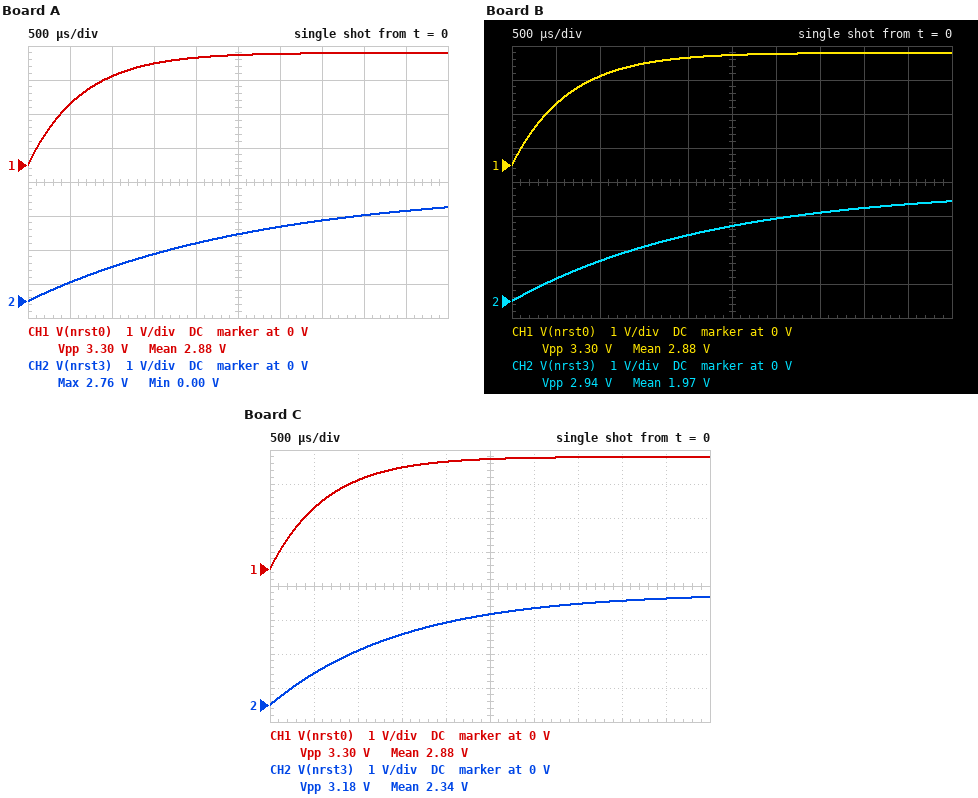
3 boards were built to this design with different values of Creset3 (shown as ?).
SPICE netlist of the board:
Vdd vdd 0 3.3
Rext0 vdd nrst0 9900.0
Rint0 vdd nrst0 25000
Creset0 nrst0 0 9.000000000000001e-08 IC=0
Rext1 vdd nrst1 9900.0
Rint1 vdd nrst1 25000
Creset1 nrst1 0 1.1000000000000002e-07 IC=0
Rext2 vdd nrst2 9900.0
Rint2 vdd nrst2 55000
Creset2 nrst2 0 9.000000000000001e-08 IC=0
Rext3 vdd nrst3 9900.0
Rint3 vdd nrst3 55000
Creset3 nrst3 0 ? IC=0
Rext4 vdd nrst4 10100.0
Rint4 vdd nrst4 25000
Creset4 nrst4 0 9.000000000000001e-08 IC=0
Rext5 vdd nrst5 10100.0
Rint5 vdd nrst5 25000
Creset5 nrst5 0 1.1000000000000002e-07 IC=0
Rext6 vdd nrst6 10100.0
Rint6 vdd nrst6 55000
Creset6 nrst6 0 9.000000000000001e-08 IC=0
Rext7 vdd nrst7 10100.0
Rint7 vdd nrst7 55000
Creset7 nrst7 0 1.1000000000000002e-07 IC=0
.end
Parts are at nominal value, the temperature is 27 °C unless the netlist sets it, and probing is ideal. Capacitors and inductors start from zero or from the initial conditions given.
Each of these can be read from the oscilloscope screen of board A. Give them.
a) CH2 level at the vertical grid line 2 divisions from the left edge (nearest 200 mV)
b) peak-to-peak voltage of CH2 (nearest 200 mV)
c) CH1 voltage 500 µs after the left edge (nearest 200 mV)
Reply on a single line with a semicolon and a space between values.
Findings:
1.0 V; 2.8 V; 1.8 V
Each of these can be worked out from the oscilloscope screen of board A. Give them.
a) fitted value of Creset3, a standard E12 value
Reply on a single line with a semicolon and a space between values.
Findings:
330 nF
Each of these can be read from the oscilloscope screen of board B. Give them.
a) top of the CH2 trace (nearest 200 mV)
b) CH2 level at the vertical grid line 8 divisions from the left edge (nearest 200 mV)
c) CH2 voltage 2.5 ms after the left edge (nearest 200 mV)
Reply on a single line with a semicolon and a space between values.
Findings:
3.0 V; 2.8 V; 2.2 V
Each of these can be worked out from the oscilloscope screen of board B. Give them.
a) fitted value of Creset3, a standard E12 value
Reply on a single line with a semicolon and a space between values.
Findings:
270 nF
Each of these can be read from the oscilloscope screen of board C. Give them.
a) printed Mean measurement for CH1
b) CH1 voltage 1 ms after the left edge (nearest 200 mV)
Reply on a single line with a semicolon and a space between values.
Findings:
2.88 V; 2.6 V
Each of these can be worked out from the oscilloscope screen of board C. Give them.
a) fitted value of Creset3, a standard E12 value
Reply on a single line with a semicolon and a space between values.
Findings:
180 nF
